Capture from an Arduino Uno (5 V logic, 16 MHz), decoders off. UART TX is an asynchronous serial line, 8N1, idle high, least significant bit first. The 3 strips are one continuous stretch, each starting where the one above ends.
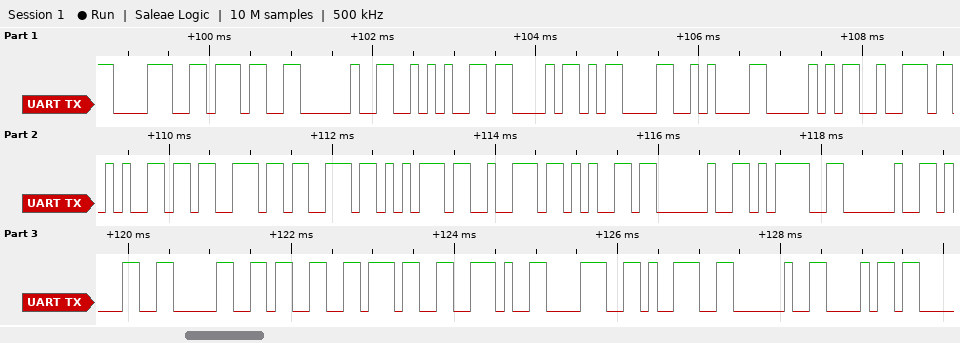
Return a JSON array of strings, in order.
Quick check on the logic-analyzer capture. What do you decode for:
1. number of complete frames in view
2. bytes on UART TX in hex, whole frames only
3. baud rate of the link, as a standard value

["27", "38 37 20 2A 43 0D 0A 50 72 65 73 73 75 72 65 20 3D 20 31 30 33 37 2E 38 39 20 68", "9600 baud"]
